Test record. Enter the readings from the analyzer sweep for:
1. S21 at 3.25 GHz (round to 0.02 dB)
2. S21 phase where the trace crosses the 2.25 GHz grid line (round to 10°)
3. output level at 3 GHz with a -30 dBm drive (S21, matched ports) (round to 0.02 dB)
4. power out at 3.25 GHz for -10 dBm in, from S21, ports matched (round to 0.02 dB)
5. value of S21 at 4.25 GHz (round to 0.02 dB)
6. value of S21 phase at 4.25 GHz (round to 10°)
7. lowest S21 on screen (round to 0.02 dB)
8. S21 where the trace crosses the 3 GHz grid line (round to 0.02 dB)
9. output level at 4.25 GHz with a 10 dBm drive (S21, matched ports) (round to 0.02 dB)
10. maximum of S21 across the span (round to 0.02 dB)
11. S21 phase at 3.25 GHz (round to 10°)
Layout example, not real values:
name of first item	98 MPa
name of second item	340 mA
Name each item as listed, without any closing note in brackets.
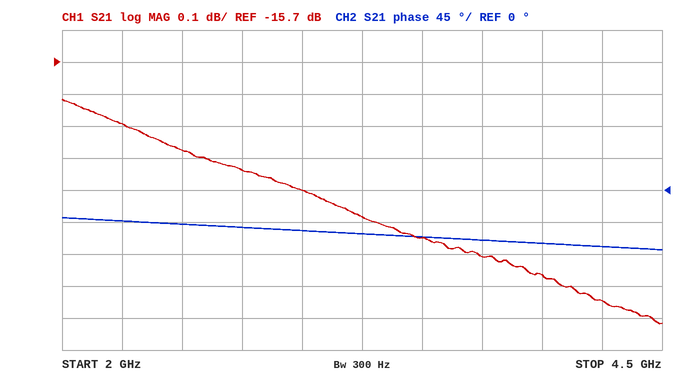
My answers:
S21 at 3.25 GHz	-16.18 dB
S21 phase where the trace crosses the 2.25 GHz grid line	-40°
output level at 3 GHz with a -30 dBm drive (S21, matched ports)	-46.10 dBm
power out at 3.25 GHz for -10 dBm in, from S21, ports matched	-26.18 dBm
value of S21 at 4.25 GHz	-16.44 dB
value of S21 phase at 4.25 GHz	-80°
lowest S21 on screen	-16.52 dB
S21 where the trace crosses the 3 GHz grid line	-16.10 dB
output level at 4.25 GHz with a 10 dBm drive (S21, matched ports)	-6.44 dBm
maximum of S21 across the span	-15.82 dB
S21 phase at 3.25 GHz	-60°
